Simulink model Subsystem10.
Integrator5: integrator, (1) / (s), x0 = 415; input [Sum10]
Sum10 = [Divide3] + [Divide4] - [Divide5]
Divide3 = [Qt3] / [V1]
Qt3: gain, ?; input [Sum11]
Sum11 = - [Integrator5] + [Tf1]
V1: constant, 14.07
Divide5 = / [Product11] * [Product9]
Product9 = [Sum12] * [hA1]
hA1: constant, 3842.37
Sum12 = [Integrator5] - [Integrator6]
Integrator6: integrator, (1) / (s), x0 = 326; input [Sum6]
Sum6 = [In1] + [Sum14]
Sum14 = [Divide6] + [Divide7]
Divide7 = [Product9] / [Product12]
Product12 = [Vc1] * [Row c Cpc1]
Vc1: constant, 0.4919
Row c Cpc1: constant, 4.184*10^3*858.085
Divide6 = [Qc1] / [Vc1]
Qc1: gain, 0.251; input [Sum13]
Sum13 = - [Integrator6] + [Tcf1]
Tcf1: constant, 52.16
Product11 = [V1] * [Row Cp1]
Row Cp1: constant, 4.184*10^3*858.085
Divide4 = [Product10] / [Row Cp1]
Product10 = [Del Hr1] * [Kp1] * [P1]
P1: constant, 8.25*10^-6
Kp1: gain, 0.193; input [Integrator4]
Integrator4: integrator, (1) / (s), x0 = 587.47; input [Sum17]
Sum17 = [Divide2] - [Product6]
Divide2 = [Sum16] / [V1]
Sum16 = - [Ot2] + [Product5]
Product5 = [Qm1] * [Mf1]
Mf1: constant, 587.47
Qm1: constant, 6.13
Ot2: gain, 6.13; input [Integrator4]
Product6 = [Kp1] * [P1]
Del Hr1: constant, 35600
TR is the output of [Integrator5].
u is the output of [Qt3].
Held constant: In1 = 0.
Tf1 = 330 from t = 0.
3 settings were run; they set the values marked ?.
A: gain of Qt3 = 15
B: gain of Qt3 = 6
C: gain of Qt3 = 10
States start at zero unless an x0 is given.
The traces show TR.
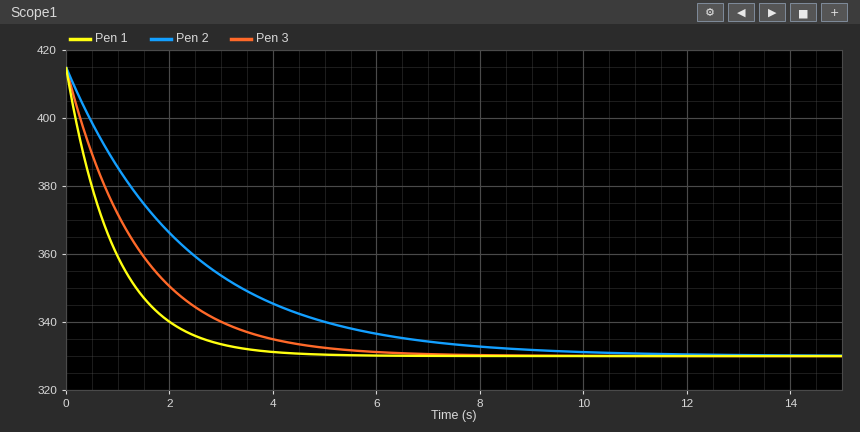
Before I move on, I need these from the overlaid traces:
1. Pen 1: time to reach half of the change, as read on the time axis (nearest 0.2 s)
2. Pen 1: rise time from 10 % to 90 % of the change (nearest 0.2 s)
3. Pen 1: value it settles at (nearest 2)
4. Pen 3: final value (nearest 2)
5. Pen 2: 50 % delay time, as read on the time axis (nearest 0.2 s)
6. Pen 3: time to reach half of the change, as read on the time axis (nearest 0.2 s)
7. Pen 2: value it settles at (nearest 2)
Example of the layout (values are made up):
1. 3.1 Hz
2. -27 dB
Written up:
1. 0.6 s
2. 2.0 s
3. 330
4. 330
5. 1.6 s
6. 1.0 s
7. 330
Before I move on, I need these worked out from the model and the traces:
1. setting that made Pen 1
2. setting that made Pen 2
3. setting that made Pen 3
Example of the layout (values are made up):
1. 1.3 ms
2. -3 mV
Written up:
1. A
2. B
3. C
